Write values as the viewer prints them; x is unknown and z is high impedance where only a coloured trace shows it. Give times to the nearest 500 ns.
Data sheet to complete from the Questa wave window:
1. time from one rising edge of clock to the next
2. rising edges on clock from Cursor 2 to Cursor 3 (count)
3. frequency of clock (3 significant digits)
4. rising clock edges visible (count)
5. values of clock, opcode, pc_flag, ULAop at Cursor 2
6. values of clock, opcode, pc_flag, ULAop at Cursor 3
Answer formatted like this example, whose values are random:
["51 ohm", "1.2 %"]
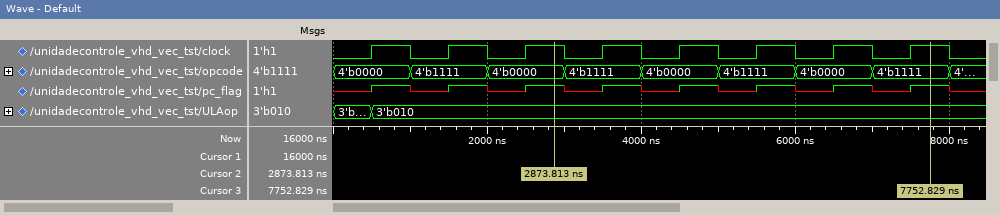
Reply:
["1000 ns", "5", "1.00 MHz", "8", "clock=1, opcode=4'b0000, pc_flag=1, ULAop=3'b010", "clock=1, opcode=4'b1111, pc_flag=1, ULAop=3'b010"]
